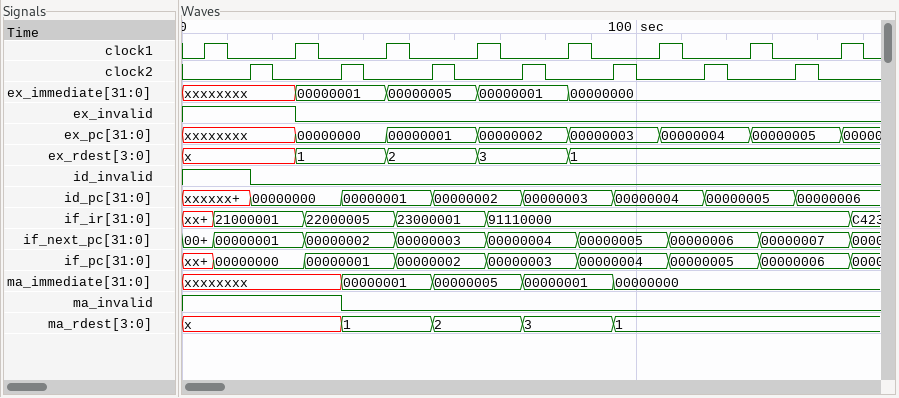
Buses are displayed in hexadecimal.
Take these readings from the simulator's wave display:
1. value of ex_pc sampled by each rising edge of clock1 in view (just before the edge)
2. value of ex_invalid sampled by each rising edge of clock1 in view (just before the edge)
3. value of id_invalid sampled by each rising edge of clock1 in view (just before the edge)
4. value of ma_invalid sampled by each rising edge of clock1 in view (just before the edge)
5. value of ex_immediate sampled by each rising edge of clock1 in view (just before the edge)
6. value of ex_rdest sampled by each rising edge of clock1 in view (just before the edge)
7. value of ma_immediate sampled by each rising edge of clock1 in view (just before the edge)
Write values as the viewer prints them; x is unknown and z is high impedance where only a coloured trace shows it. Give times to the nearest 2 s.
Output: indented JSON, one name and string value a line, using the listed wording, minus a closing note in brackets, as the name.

{
  "value of ex_pc sampled by each rising edge of clock1 in view": "xxxxxxxx, xxxxxxxx, 00000000, 00000001, 00000002, 00000003, 00000004, 00000005",
  "value of ex_invalid sampled by each rising edge of clock1 in view": "1 1 0 0 0 0 0 0",
  "value of id_invalid sampled by each rising edge of clock1 in view": "1 0 0 0 0 0 0 0",
  "value of ma_invalid sampled by each rising edge of clock1 in view": "1 1 0 0 0 0 0 0",
  "value of ex_immediate sampled by each rising edge of clock1 in view": "xxxxxxxx, xxxxxxxx, 00000001, 00000005, 00000001, 00000000, 00000000, 00000000",
  "value of ex_rdest sampled by each rising edge of clock1 in view": "x, x, 1, 2, 3, 1, 1, 1",
  "value of ma_immediate sampled by each rising edge of clock1 in view": "xxxxxxxx, xxxxxxxx, 00000001, 00000005, 00000001, 00000000, 00000000, 00000000"
}
